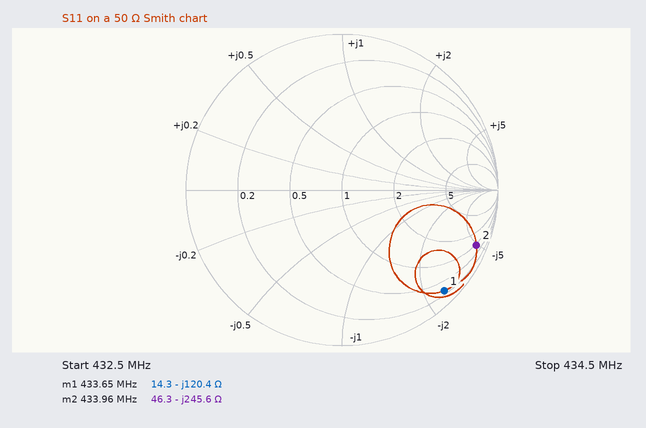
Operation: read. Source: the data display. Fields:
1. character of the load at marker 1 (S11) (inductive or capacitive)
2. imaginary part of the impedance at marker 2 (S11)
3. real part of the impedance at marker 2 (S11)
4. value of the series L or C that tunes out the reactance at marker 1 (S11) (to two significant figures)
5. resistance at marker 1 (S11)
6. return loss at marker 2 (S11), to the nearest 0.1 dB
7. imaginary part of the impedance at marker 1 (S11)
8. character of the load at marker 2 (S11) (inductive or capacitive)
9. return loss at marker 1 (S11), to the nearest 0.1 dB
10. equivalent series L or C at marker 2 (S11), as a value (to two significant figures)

capacitive
-245.6 Ω
46.3 Ω
44 nH
14.3 Ω
0.6 dB
-120.4 Ω
capacitive
0.7 dB
1.5 pF
